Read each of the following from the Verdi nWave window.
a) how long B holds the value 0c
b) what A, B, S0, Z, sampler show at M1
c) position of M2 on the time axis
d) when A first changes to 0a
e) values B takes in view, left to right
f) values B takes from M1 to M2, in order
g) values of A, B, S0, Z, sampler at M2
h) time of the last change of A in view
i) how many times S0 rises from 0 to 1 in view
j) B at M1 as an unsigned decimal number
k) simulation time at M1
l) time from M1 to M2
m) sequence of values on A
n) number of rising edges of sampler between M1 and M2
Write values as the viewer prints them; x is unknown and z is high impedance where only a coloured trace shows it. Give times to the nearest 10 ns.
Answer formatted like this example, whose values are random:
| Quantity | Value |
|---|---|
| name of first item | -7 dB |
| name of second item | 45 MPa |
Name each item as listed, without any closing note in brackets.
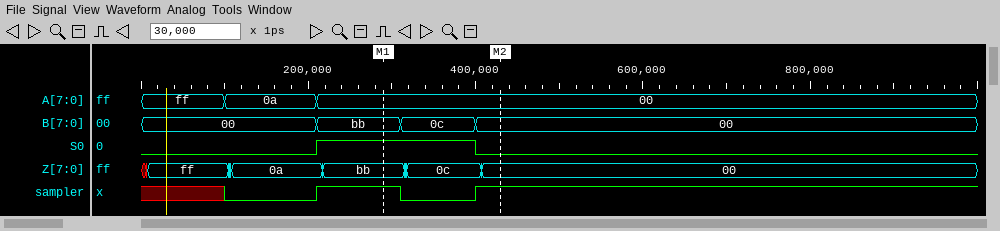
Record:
| Quantity | Value |
|---|---|
| how long B holds the value 0c | 90 ns |
| what A, B, S0, Z, sampler show at M1 | A=00, B=bb, S0=1, Z=bb, sampler=1 |
| position of M2 on the time axis | 430 ns |
| when A first changes to 0a | 100 ns |
| values B takes in view, left to right | 00, bb, 0c, 00 |
| values B takes from M1 to M2, in order | bb, 0c, 00 |
| values of A, B, S0, Z, sampler at M2 | A=00, B=00, S0=0, Z=00, sampler=1 |
| time of the last change of A in view | 210 ns |
| how many times S0 rises from 0 to 1 in view | 1 |
| B at M1 as an unsigned decimal number | 187 |
| simulation time at M1 | 290 ns |
| time from M1 to M2 | 140 ns |
| sequence of values on A | ff, 0a, 00 |
| number of rising edges of sampler between M1 and M2 | 1 |
